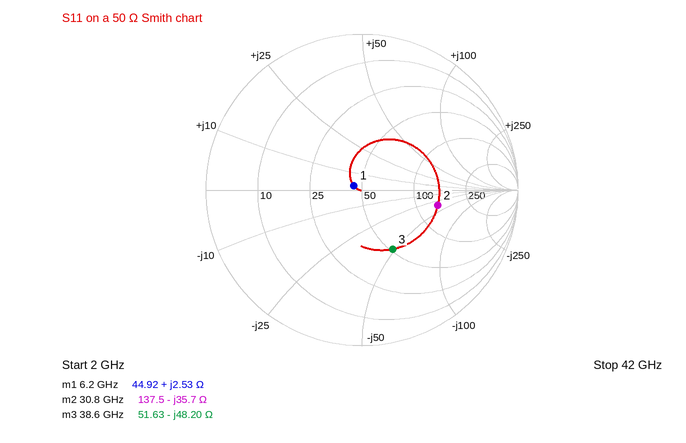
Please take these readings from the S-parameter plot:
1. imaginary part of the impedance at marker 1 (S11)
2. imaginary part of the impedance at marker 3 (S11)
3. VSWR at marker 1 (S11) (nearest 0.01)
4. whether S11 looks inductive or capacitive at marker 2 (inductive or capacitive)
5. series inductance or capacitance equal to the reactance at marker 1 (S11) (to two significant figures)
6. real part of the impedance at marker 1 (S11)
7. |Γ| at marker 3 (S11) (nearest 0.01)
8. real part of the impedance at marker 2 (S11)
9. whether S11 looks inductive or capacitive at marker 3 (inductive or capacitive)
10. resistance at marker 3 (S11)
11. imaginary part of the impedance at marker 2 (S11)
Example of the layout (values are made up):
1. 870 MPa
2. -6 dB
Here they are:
1. +2.53 Ω
2. -48.20 Ω
3. 1.13
4. capacitive
5. 65 pH
6. 44.92 Ω
7. 0.43
8. 137.5 Ω
9. capacitive
10. 51.63 Ω
11. -35.7 Ω
